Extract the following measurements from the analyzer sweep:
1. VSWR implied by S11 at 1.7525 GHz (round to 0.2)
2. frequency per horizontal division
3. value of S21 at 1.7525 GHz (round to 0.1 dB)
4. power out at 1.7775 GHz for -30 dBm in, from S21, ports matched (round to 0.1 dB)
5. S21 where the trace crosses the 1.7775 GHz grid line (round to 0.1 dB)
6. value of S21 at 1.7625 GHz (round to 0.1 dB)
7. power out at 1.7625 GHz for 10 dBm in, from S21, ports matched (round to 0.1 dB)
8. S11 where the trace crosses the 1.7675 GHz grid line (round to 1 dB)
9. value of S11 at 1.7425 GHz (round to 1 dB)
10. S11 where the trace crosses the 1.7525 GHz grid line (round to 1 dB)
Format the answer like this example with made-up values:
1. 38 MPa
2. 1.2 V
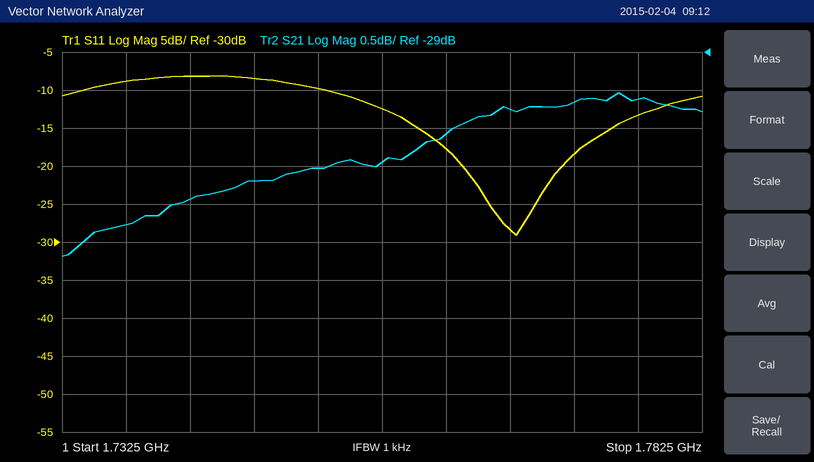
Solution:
1. 2.0
2. 5 MHz
3. -30.5 dB
4. -59.6 dBm
5. -29.6 dB
6. -30.1 dB
7. -20.1 dBm
8. -28 dB
9. -8 dB
10. -10 dB
